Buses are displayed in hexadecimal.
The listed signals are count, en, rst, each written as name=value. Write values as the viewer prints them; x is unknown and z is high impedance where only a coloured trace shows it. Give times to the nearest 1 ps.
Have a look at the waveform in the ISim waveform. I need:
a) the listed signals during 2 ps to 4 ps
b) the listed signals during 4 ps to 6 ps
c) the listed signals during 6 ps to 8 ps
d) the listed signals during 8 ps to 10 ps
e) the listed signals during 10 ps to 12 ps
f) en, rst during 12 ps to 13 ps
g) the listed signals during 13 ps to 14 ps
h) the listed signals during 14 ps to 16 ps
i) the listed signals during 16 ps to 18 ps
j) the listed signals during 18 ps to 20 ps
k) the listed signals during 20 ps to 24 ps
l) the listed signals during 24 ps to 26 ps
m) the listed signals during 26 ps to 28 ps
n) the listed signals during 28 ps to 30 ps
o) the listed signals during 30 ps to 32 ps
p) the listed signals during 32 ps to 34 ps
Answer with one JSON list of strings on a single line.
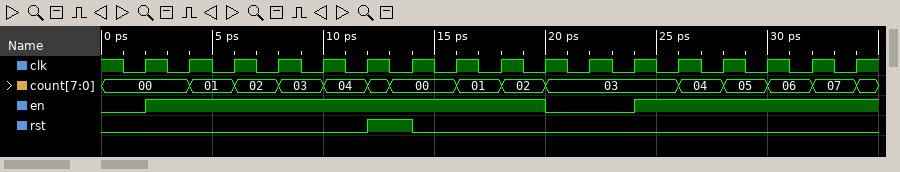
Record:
["count=00, en=1, rst=0", "count=01, en=1, rst=0", "count=02, en=1, rst=0", "count=03, en=1, rst=0", "count=04, en=1, rst=0", "en=1, rst=1", "count=00, en=1, rst=1", "count=00, en=1, rst=0", "count=01, en=1, rst=0", "count=02, en=1, rst=0", "count=03, en=0, rst=0", "count=03, en=1, rst=0", "count=04, en=1, rst=0", "count=05, en=1, rst=0", "count=06, en=1, rst=0", "count=07, en=1, rst=0"]
